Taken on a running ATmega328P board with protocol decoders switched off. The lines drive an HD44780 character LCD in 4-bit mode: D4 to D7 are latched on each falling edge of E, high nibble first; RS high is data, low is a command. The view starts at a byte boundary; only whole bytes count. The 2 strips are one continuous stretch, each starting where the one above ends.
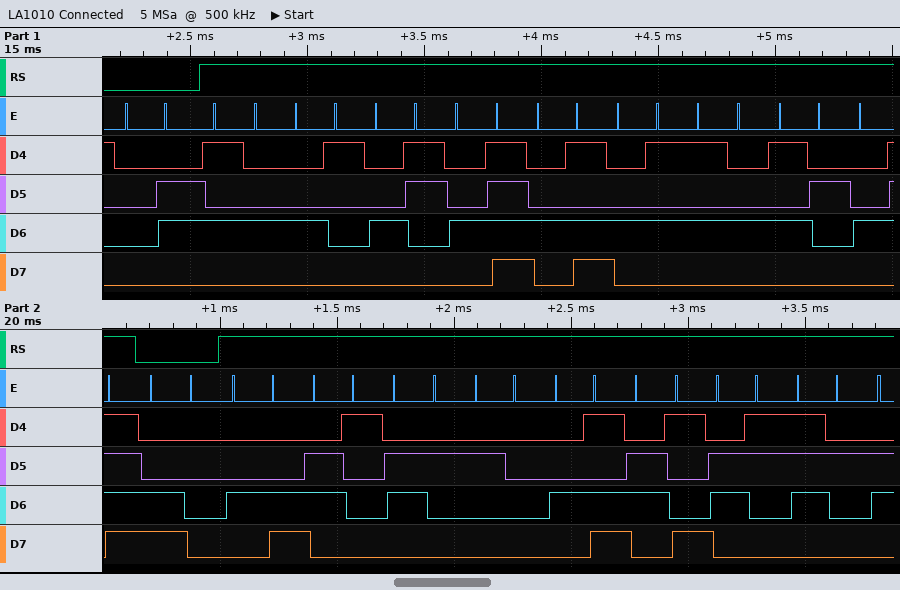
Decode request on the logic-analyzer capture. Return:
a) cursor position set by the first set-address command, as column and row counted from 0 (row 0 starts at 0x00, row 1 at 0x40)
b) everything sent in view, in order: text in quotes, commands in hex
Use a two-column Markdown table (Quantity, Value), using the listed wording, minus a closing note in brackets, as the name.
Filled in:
| Quantity | Value |
|---|---|
| cursor position set by the first set-address command, as column and row counted from 0 | column 0, row 1 |
| everything sent in view, in order: text in quotes, commands in hex | 0x06 "TACOMETRO" 0xC0 "Lab Micr" |
